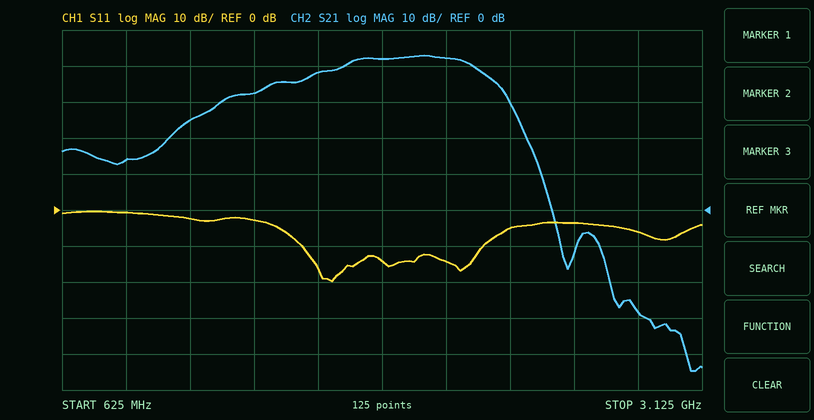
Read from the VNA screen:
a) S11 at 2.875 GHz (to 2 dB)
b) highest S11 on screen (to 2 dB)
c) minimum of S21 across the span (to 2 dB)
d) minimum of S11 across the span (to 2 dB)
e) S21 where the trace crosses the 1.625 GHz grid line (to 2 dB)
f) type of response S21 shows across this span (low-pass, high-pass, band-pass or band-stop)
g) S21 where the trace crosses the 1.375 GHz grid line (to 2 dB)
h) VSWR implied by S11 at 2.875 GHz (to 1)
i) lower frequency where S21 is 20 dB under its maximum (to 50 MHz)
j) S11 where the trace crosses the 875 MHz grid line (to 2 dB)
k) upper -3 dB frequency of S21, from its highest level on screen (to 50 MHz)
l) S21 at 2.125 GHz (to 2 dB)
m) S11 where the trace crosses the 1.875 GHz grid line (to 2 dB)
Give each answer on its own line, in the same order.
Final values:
-6 dB
0 dB
-44 dB
-20 dB
38 dB
band-pass
32 dB
3
1.10 GHz
0 dB
2.25 GHz
42 dB
-14 dB
